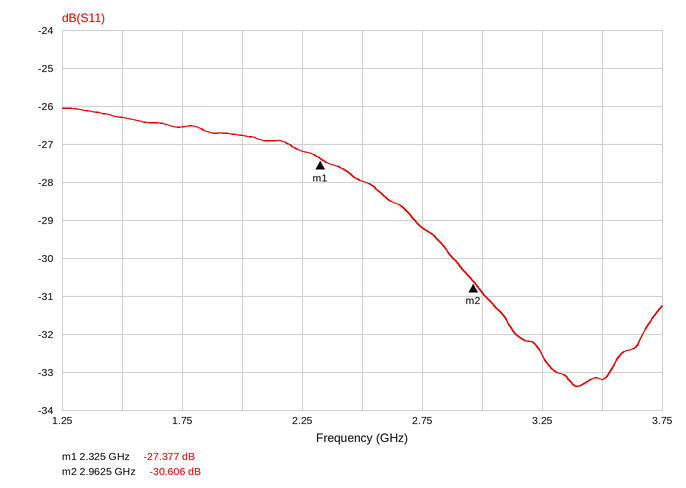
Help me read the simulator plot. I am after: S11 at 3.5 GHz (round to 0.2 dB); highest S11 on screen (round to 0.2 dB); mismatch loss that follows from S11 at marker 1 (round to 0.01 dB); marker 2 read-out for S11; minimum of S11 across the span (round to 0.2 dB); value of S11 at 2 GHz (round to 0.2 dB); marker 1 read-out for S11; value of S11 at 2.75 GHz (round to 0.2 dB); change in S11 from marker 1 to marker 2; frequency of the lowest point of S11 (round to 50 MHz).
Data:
-33.2 dB
-26.0 dB
0.01 dB
-30.606 dB
-33.4 dB
-26.8 dB
-27.377 dB
-29.2 dB
-3.229 dB
3.40 GHz
